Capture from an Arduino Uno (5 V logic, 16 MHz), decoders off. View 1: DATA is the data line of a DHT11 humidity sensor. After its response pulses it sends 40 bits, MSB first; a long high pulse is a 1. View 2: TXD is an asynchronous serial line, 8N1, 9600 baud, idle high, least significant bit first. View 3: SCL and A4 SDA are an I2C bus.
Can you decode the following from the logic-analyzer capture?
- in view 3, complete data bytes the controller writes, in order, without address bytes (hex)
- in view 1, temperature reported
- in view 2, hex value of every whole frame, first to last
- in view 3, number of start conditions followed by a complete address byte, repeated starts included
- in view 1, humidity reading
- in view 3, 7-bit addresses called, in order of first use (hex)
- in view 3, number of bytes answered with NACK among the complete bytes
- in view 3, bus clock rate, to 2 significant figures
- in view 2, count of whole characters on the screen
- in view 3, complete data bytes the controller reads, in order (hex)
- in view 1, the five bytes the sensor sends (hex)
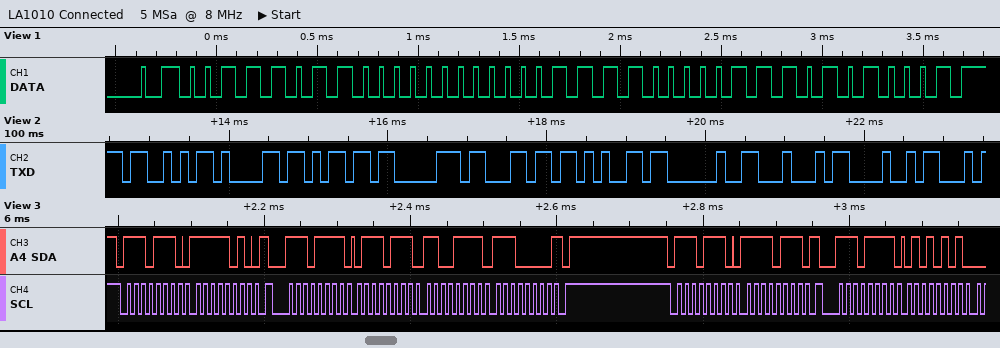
FA F7
15.7 °C
53 61 6D 70 6C 65 20 44 48
4
59 %
0x77
1
100 kHz
9
77 CF E0 55
3B 00 0F 07 51
